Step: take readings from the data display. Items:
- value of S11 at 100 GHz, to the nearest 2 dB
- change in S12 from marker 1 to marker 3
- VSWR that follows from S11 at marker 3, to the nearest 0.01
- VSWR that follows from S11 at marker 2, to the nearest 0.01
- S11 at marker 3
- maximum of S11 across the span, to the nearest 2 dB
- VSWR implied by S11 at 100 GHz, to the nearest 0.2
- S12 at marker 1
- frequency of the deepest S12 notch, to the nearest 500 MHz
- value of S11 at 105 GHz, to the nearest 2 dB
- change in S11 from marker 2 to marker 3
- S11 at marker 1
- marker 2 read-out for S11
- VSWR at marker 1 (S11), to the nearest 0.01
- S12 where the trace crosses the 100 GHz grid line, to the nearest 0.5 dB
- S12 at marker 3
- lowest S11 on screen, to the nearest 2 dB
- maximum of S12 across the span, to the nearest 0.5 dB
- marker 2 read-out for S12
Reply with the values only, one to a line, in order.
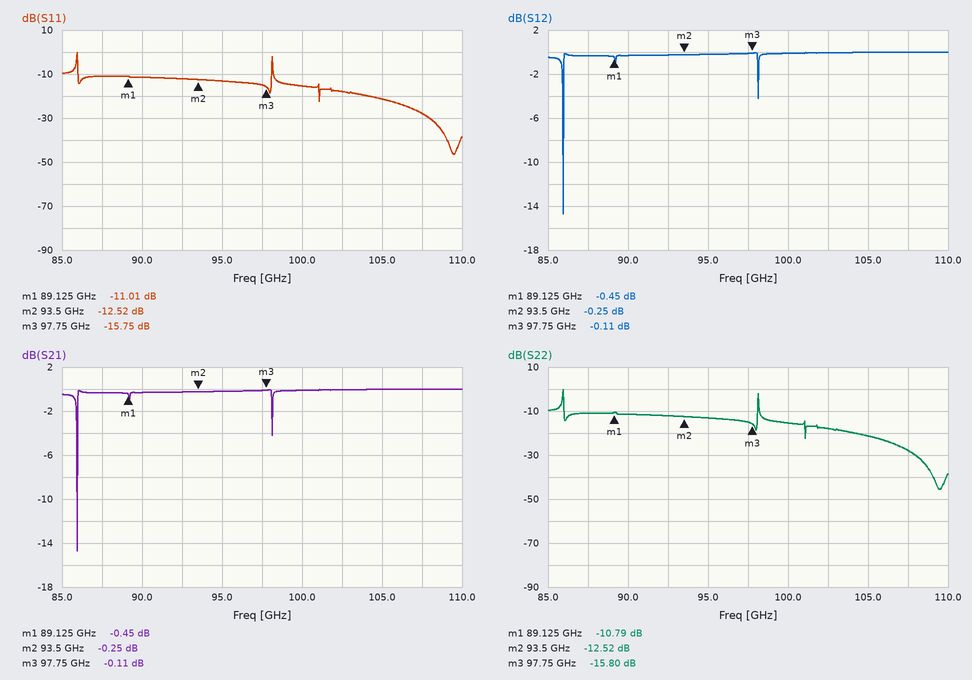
-16 dB
0.34 dB
1.39
1.62
-15.75 dB
0 dB
1.4
-0.45 dB
86.0 GHz
-22 dB
-3.23 dB
-11.01 dB
-12.52 dB
1.78
0.0 dB
-0.11 dB
-46 dB
0.0 dB
-0.25 dB
